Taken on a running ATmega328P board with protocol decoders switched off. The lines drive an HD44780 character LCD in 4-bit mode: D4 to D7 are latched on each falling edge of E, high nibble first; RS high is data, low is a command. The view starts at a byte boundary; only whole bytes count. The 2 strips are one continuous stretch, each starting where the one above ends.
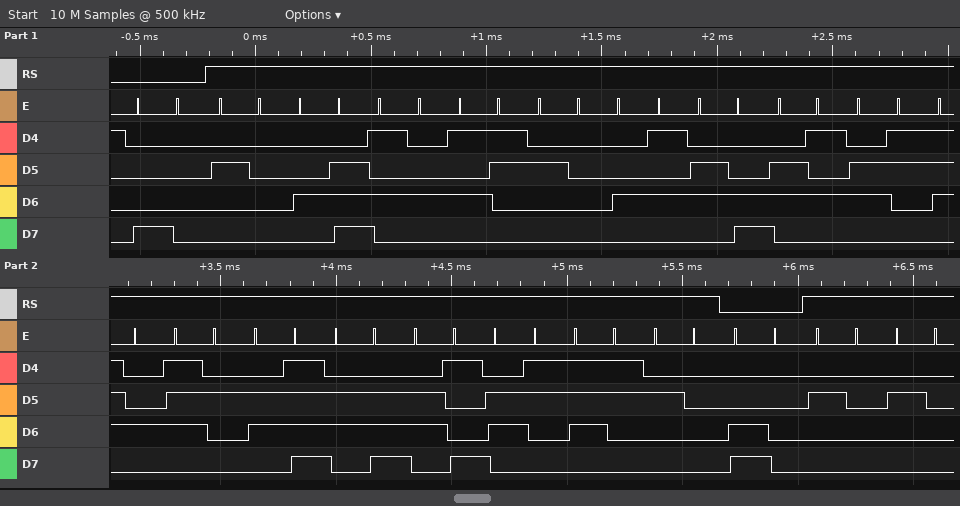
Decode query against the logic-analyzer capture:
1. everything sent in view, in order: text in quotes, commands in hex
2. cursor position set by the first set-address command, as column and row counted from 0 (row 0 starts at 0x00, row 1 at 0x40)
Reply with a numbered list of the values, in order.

1. 0x80 " NTS Electronics " 0xC0 "  "
2. column 0, row 0
